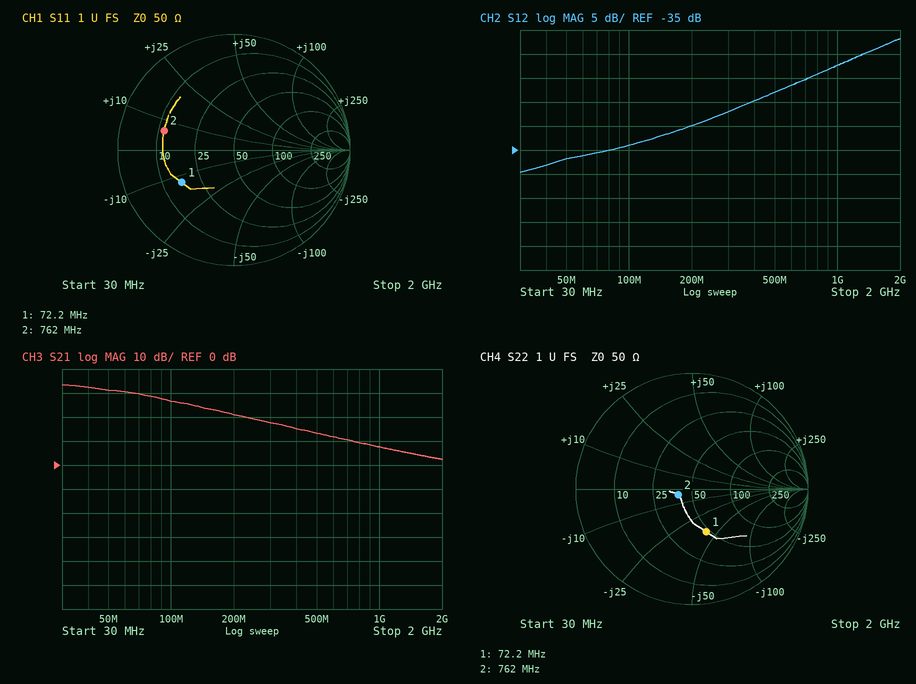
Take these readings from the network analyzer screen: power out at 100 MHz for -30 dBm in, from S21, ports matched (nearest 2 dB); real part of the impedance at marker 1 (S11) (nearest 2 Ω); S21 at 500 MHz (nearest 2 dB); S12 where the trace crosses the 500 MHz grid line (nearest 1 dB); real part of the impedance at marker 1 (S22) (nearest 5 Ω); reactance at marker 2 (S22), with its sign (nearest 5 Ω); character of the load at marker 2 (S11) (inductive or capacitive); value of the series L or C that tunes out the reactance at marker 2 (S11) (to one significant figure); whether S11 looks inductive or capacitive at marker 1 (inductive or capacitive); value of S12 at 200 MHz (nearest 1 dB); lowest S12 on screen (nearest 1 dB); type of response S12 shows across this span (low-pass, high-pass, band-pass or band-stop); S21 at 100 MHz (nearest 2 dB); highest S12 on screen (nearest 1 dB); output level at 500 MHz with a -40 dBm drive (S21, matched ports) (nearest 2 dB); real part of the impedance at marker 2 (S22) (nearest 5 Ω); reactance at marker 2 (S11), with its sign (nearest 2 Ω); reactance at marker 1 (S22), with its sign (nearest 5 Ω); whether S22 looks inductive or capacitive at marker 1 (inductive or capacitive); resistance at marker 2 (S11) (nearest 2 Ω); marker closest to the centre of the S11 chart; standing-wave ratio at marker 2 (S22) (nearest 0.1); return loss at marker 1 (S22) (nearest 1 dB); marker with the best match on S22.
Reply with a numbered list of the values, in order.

1. -4 dBm
2. 16 Ω
3. 14 dB
4. -23 dB
5. 45 Ω
6. -5 Ω
7. inductive
8. 30 pF
9. capacitive
10. -30 dB
11. -40 dB
12. high-pass
13. 26 dB
14. -12 dB
15. -26 dBm
16. 40 Ω
17. +6 Ω
18. -40 Ω
19. capacitive
20. 12 Ω
21. marker 1
22. 1.3
23. 8 dB
24. marker 2
